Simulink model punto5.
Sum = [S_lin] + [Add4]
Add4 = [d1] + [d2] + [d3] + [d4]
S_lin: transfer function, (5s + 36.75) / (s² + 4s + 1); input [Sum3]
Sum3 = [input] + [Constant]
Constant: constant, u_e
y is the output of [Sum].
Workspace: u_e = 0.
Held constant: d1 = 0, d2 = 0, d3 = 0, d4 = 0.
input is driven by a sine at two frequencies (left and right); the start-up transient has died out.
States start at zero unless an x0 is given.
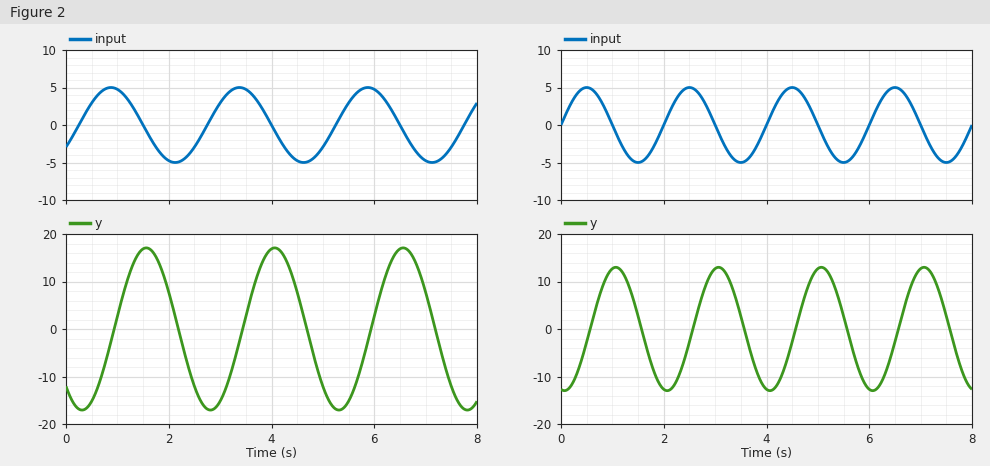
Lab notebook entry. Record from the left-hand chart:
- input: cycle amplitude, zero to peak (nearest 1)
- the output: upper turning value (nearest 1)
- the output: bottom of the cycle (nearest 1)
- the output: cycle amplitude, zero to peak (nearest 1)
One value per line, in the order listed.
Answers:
5
17
-17
17
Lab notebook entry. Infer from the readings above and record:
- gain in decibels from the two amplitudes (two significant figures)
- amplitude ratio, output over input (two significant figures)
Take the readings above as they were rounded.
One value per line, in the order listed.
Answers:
11 dB
3.4
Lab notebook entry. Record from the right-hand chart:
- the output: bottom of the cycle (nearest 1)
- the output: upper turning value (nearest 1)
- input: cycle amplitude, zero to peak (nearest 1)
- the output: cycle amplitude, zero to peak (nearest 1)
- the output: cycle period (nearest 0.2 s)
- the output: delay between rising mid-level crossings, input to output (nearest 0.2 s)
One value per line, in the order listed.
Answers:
-13
13
5
13
2.0 s
0.6 s
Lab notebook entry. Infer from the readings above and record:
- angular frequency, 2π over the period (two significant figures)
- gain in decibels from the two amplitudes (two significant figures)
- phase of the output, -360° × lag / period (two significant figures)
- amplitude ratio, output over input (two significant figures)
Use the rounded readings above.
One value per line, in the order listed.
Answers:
3.1 rad/s
8.3 dB
-110°
2.6
